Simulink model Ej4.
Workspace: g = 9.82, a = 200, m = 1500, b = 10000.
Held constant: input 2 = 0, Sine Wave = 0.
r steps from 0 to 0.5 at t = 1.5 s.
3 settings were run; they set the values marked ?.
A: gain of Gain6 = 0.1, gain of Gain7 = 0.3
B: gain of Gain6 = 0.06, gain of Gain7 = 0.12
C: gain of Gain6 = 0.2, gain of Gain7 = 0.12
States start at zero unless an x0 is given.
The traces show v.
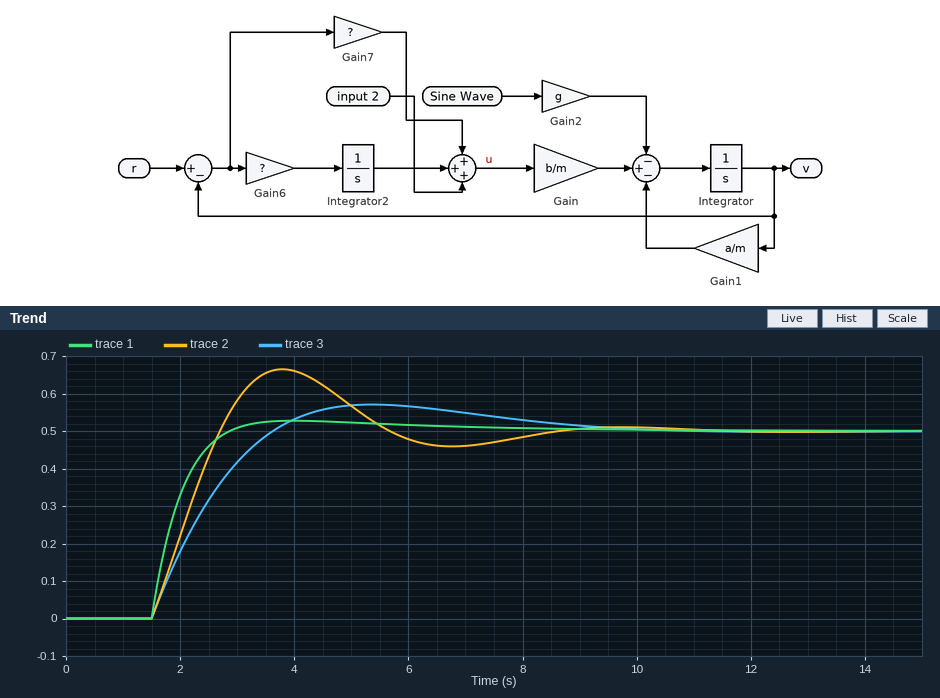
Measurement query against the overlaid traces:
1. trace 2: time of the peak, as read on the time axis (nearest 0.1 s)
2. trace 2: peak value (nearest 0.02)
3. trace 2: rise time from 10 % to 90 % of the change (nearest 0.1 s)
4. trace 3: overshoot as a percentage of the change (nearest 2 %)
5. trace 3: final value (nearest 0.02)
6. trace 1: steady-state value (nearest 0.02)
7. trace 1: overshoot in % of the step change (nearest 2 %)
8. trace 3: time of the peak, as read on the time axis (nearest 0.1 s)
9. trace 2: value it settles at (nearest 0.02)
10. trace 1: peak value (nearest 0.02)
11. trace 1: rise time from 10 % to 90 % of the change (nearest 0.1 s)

3.8 s
0.66
0.9 s
14 %
0.50
0.50
6 %
5.4 s
0.50
0.52
0.9 s
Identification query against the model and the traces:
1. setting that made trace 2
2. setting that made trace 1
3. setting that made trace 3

C
A
B
